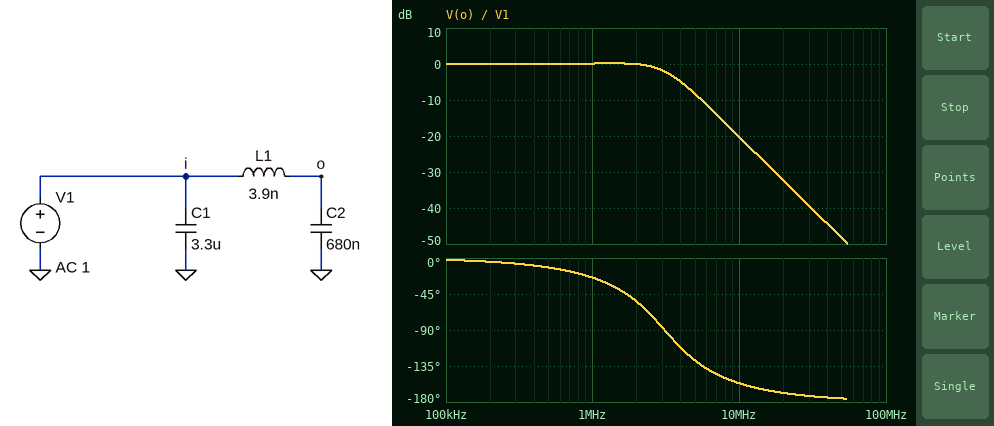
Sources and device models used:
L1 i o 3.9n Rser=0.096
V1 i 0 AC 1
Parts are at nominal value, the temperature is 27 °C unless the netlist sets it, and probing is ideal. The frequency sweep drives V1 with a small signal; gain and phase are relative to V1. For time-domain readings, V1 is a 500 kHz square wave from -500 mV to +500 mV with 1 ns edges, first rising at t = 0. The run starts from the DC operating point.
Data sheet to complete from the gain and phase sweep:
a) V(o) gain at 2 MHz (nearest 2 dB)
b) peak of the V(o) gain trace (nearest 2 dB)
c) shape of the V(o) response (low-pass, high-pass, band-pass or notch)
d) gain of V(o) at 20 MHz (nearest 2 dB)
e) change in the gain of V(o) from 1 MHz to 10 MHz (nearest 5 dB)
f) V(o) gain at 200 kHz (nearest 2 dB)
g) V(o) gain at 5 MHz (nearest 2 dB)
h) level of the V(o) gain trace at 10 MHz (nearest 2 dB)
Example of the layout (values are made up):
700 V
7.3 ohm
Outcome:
0 dB
0 dB
low-pass
-32 dB
-20 dB
0 dB
-8 dB
-20 dB
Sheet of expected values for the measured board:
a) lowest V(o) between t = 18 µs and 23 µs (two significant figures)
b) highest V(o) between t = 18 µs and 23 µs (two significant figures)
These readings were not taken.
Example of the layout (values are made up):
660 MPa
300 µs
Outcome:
-580 mV
580 mV
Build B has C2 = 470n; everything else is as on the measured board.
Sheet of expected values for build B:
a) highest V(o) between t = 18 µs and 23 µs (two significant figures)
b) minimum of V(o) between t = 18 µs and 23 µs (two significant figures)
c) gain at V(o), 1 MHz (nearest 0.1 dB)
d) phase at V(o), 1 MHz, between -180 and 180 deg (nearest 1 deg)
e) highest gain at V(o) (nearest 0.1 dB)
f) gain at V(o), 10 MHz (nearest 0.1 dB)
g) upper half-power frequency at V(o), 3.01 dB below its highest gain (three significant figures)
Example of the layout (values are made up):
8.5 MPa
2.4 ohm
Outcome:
640 mV
-640 mV
0.3 dB
-17 deg
1.0 dB
-16.7 dB
4.30 MHz
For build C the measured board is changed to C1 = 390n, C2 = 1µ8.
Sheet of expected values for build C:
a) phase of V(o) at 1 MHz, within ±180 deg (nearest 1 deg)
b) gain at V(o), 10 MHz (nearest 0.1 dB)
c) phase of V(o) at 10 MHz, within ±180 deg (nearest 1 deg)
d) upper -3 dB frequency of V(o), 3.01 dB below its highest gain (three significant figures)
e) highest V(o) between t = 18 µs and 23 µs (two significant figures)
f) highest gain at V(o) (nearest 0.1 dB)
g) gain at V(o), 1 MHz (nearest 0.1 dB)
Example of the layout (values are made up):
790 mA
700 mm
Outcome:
-56 deg
-29.2 dB
-158 deg
1.17 MHz
500 mV
0 dB
-2.3 dB
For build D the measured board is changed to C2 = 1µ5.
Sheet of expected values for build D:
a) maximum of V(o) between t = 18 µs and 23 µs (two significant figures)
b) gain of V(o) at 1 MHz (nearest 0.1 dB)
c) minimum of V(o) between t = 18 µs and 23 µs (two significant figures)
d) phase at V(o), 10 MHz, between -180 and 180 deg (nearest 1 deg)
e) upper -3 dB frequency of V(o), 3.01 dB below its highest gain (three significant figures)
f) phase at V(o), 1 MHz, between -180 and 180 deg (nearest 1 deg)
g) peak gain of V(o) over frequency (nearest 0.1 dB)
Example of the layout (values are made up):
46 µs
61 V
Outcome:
500 mV
-1.5 dB
-500 mV
-158 deg
1.46 MHz
-50 deg
0 dB
